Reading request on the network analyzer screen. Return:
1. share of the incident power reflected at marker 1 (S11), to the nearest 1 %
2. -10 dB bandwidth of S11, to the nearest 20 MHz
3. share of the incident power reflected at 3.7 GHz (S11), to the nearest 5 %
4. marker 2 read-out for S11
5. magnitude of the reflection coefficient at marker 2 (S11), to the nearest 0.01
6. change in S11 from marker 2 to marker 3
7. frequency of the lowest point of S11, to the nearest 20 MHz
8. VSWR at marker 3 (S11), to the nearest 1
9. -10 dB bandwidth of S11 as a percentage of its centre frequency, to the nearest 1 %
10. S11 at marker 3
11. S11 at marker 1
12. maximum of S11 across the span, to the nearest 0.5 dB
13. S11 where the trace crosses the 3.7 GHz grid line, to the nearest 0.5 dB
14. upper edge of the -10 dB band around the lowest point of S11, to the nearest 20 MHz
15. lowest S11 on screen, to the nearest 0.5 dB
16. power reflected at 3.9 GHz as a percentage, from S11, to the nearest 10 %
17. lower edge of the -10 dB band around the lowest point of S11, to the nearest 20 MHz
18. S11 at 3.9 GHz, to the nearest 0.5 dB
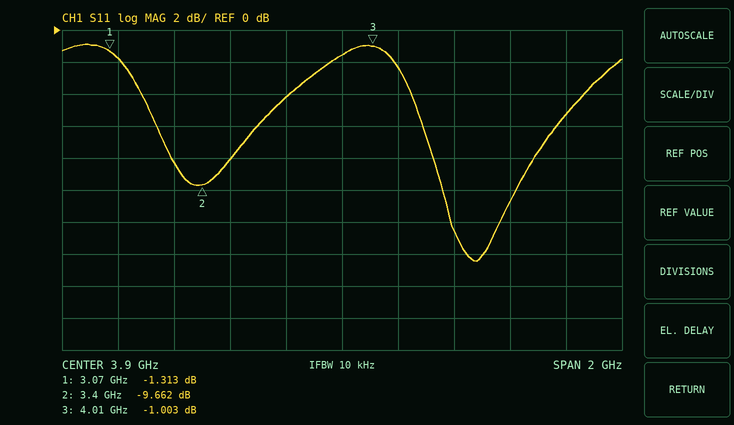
74 %
260 MHz
40 %
-9.662 dB
0.33
8.659 dB
4.38 GHz
17
6 %
-1.003 dB
-1.313 dB
-1.0 dB
-4.0 dB
4.52 GHz
-14.5 dB
70 %
4.26 GHz
-1.5 dB
